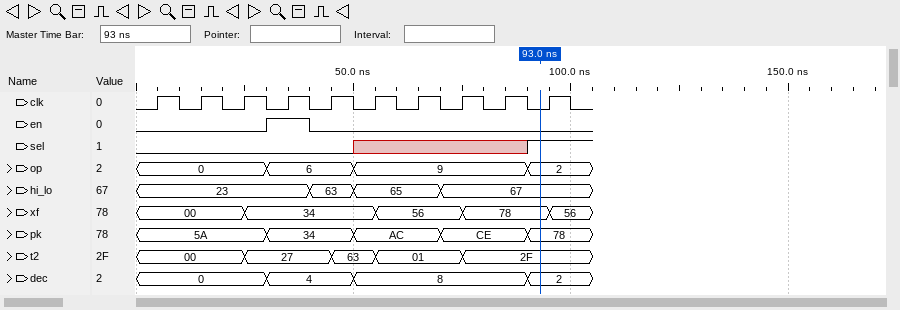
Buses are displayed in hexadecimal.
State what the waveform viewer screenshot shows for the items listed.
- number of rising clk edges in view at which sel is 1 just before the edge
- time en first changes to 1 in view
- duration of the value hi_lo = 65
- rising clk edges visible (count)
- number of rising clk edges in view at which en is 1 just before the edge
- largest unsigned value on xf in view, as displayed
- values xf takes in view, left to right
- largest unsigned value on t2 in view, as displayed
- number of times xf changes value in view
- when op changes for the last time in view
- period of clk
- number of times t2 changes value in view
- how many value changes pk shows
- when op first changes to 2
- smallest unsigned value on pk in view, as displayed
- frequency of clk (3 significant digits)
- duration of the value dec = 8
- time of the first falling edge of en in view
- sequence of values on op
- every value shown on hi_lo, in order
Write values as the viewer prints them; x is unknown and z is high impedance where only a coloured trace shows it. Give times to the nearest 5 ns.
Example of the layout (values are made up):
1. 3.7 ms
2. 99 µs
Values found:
1. 1
2. 30 ns
3. 20 ns
4. 10
5. 1
6. 78
7. 00, 34, 56, 78, 56
8. 63
9. 4
10. 90 ns
11. 10 ns
12. 4
13. 4
14. 90 ns
15. 34
16. 100 MHz
17. 40 ns
18. 40 ns
19. 0, 6, 9, 2
20. 23, 63, 65, 67
